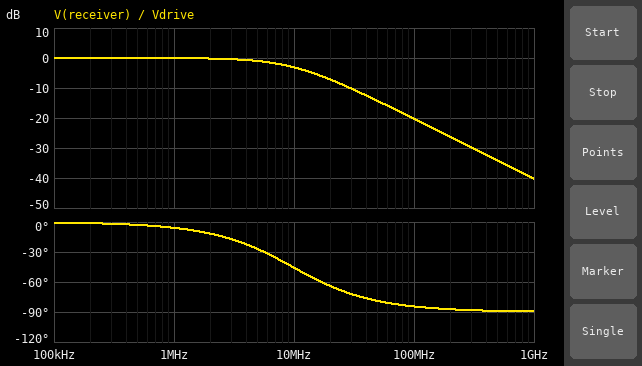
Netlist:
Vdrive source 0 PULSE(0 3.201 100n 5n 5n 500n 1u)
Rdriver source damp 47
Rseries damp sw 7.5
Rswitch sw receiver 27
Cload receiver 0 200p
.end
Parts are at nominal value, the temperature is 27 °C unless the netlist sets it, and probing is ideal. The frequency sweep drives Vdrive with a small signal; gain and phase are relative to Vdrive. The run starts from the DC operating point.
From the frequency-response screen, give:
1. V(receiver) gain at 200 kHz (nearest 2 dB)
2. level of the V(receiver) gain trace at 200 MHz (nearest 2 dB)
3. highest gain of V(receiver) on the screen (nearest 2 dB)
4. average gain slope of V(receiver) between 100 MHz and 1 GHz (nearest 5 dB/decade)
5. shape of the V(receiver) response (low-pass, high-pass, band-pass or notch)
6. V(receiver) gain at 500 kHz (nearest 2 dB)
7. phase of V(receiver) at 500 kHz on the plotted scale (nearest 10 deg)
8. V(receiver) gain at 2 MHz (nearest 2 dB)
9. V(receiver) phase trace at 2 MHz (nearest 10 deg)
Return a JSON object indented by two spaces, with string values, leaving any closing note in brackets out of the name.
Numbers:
{
  "V(receiver) gain at 200 kHz": "0 dB",
  "level of the V(receiver) gain trace at 200 MHz": "-26 dB",
  "highest gain of V(receiver) on the screen": "0 dB",
  "average gain slope of V(receiver) between 100 MHz and 1 GHz": "-20 dB/decade",
  "shape of the V(receiver) response": "low-pass",
  "V(receiver) gain at 500 kHz": "0 dB",
  "phase of V(receiver) at 500 kHz on the plotted scale": "0 deg",
  "V(receiver) gain at 2 MHz": "0 dB",
  "V(receiver) phase trace at 2 MHz": "-10 deg"
}
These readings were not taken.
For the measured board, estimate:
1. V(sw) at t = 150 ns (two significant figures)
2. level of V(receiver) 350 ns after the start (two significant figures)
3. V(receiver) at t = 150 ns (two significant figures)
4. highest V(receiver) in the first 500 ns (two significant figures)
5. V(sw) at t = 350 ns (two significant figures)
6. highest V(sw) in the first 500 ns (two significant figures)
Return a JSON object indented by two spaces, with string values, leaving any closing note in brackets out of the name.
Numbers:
{
  "V(sw) at t = 150 ns": "3.1 V",
  "level of V(receiver) 350 ns after the start": "3.2 V",
  "V(receiver) at t = 150 ns": "3.0 V",
  "highest V(receiver) in the first 500 ns": "3.2 V",
  "V(sw) at t = 350 ns": "3.2 V",
  "highest V(sw) in the first 500 ns": "3.2 V"
}
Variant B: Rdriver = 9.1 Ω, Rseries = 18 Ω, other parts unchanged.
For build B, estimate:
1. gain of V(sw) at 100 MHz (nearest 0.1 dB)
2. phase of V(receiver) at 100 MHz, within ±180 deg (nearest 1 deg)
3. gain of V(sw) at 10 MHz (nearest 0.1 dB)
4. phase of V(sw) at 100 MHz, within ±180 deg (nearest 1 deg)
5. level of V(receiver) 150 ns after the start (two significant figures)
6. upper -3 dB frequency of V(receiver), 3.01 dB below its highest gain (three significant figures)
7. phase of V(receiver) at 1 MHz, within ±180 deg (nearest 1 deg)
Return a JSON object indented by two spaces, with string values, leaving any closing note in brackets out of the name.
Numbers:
{
  "gain of V(sw) at 100 MHz": "-5.8 dB",
  "phase of V(receiver) at 100 MHz, within ±180 deg": "-82 deg",
  "gain of V(sw) at 10 MHz": "-1.2 dB",
  "phase of V(sw) at 100 MHz, within ±180 deg": "-8 deg",
  "level of V(receiver) 150 ns after the start": "3.2 V",
  "upper -3 dB frequency of V(receiver), 3.01 dB below its highest gain": "14.7 MHz",
  "phase of V(receiver) at 1 MHz, within ±180 deg": "-4 deg"
}
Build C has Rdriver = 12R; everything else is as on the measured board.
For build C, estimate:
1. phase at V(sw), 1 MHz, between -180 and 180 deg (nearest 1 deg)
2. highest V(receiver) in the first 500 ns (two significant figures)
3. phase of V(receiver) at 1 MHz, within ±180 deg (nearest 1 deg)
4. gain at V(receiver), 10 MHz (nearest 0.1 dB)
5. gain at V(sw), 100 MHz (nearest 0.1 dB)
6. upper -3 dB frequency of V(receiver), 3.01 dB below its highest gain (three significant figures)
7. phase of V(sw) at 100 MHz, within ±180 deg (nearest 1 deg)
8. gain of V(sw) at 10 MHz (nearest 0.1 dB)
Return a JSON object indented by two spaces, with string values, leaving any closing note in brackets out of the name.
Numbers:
{
  "phase at V(sw), 1 MHz, between -180 and 180 deg": "-1 deg",
  "highest V(receiver) in the first 500 ns": "3.2 V",
  "phase of V(receiver) at 1 MHz, within ±180 deg": "-3 deg",
  "gain at V(receiver), 10 MHz": "-1.3 dB",
  "gain at V(sw), 100 MHz": "-4.5 dB",
  "upper -3 dB frequency of V(receiver), 3.01 dB below its highest gain": "17.1 MHz",
  "phase of V(sw) at 100 MHz, within ±180 deg": "-7 deg",
  "gain of V(sw) at 10 MHz": "-0.8 dB"
}
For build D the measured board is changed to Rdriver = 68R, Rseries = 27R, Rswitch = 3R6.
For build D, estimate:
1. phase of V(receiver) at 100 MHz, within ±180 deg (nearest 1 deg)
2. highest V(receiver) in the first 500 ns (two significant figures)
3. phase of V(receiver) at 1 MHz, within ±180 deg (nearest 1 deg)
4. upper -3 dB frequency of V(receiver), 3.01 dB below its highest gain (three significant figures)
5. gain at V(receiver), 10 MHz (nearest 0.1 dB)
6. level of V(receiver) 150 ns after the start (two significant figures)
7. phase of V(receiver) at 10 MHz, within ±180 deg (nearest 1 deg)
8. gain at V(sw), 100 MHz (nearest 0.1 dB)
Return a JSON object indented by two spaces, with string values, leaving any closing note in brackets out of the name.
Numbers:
{
  "phase of V(receiver) at 100 MHz, within ±180 deg": "-85 deg",
  "highest V(receiver) in the first 500 ns": "3.2 V",
  "phase of V(receiver) at 1 MHz, within ±180 deg": "-7 deg",
  "upper -3 dB frequency of V(receiver), 3.01 dB below its highest gain": "8.07 MHz",
  "gain at V(receiver), 10 MHz": "-4.0 dB",
  "level of V(receiver) 150 ns after the start": "2.9 V",
  "phase of V(receiver) at 10 MHz, within ±180 deg": "-51 deg",
  "gain at V(sw), 100 MHz": "-21.1 dB"
}
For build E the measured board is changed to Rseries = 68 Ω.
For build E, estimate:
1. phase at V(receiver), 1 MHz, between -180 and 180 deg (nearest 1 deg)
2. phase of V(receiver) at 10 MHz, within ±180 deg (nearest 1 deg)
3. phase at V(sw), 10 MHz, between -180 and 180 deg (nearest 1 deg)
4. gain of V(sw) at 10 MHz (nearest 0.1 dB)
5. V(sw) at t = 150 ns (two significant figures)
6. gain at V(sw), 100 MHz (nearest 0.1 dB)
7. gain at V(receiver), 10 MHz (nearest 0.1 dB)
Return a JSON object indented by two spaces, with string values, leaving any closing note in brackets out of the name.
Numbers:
{
  "phase at V(receiver), 1 MHz, between -180 and 180 deg": "-10 deg",
  "phase of V(receiver) at 10 MHz, within ±180 deg": "-61 deg",
  "phase at V(sw), 10 MHz, between -180 and 180 deg": "-42 deg",
  "gain of V(sw) at 10 MHz": "-5.7 dB",
  "V(sw) at t = 150 ns": "2.7 V",
  "gain at V(sw), 100 MHz": "-14.1 dB",
  "gain at V(receiver), 10 MHz": "-6.2 dB"
}
